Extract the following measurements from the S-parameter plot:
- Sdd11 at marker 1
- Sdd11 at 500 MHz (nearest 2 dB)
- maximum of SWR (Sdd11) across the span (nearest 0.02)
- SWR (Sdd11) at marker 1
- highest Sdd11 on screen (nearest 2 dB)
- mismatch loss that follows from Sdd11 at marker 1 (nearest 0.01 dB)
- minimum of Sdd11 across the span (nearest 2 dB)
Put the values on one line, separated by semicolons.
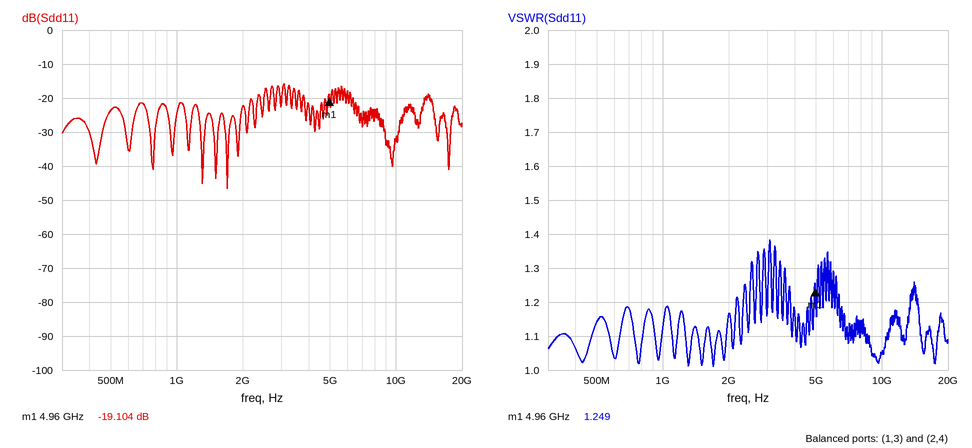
-19.104 dB; -24 dB; 1.38; 1.249; -16 dB; 0.05 dB; -46 dB
